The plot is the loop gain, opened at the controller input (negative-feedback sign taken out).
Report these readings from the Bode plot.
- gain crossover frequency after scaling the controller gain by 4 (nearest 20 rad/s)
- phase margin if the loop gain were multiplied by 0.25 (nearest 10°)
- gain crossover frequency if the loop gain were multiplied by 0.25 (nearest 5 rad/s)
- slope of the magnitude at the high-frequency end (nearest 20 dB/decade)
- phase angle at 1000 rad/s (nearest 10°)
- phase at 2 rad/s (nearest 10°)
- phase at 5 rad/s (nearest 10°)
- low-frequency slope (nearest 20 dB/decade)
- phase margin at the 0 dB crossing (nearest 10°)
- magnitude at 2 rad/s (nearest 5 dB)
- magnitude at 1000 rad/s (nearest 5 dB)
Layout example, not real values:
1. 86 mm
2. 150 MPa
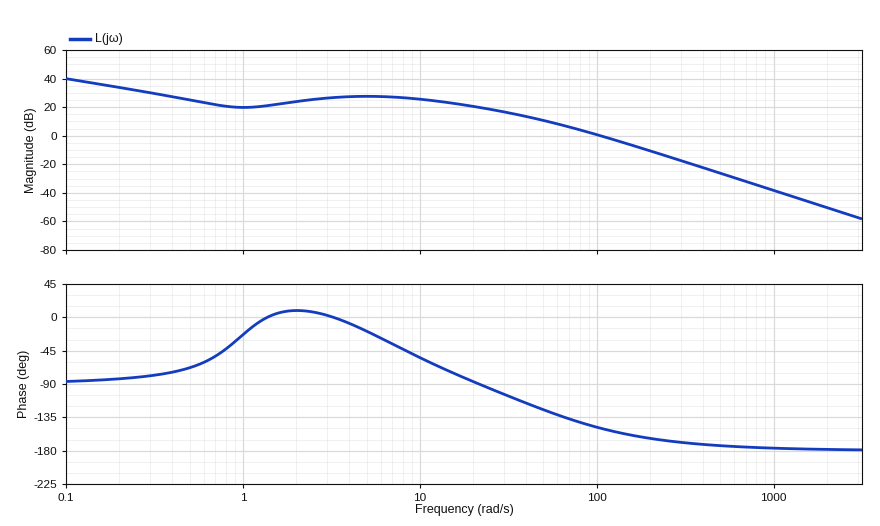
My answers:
1. 220 rad/s
2. 60°
3. 45 rad/s
4. -40 dB/decade
5. -180°
6. 10°
7. -20°
8. -20 dB/decade
9. 30°
10. 25 dB
11. -40 dB
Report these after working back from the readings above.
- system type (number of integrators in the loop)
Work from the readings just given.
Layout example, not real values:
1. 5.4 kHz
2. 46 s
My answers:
1. 1
